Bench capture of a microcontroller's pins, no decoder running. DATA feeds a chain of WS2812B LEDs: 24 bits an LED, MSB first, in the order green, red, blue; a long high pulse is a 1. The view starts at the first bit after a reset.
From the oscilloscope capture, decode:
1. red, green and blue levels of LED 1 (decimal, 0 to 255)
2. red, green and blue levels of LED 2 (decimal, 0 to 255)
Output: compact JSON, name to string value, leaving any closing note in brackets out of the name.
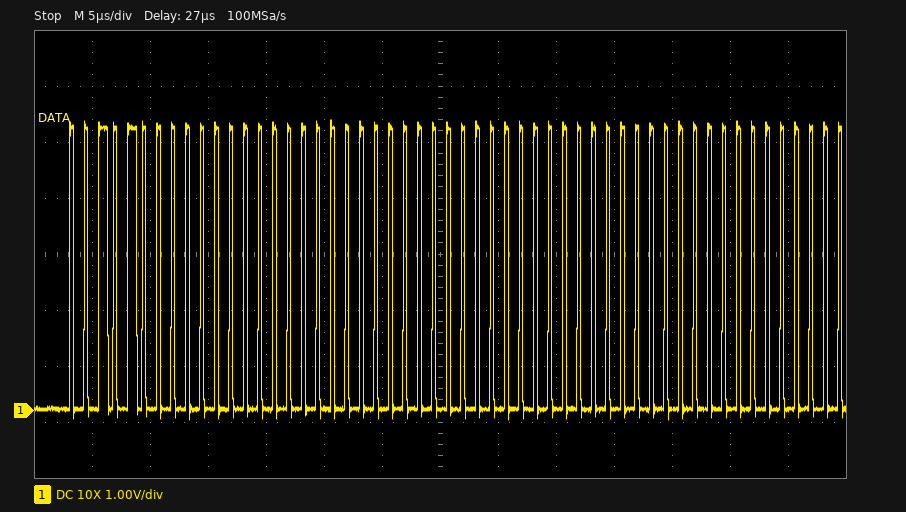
{"red, green and blue levels of LED 1": "0, 40, 0", "red, green and blue levels of LED 2": "0, 0, 0"}
